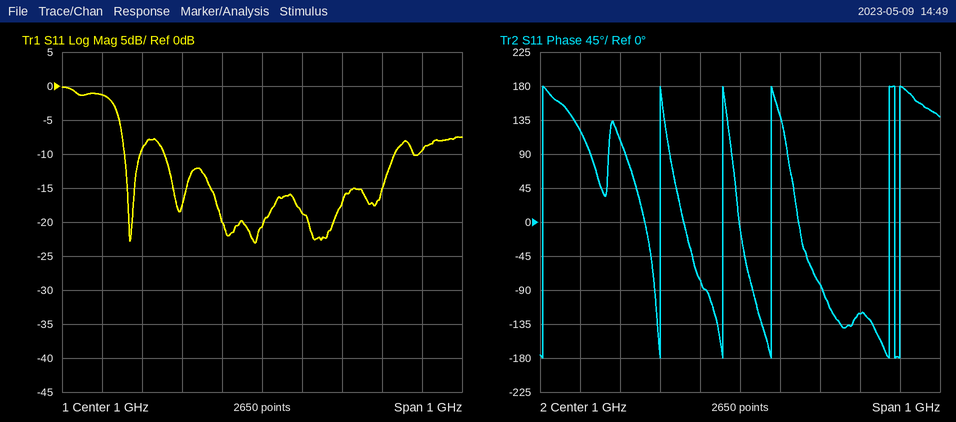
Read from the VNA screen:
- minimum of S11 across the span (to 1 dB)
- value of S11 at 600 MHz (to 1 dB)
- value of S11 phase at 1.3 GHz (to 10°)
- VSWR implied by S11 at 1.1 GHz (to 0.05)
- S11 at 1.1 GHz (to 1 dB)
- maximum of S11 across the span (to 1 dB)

-23 dB
-1 dB
-120°
1.25
-19 dB
0 dB
